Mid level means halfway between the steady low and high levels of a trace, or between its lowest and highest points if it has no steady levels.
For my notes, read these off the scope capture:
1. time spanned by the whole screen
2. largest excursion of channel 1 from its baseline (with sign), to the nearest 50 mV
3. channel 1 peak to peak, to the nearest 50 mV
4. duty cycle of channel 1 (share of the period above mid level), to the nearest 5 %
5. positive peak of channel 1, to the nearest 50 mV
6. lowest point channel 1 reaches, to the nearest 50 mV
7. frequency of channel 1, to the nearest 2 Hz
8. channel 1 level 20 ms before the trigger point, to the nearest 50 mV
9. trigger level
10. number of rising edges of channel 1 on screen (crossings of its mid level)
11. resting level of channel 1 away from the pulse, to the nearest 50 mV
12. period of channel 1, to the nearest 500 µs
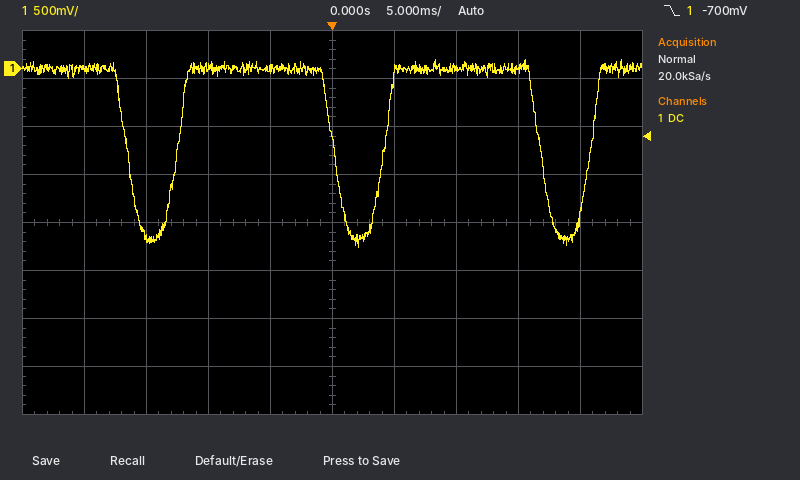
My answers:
50 ms
-1.85 V
1.95 V
75 %
100 mV
-1.85 V
60 Hz
0 mV
-700 mV
3
0 mV
16.5 ms
